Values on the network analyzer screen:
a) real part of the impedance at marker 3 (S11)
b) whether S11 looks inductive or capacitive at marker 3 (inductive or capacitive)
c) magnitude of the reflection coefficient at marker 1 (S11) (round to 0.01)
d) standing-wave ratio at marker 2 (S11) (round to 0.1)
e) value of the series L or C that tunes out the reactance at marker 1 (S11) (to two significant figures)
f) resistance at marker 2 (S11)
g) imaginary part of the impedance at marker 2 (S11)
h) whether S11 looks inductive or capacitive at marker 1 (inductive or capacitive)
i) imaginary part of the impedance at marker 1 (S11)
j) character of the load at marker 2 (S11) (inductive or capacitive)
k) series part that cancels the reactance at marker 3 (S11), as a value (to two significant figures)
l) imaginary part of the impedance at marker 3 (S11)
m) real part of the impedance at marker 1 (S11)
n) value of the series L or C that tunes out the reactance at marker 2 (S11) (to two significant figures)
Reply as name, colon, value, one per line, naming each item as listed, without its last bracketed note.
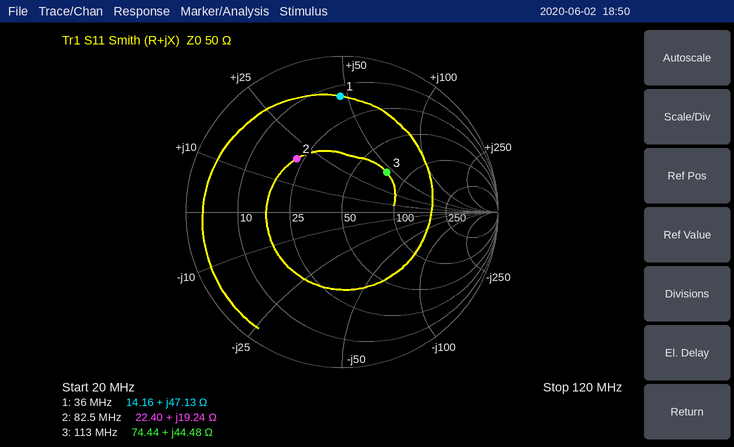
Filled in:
real part of the impedance at marker 3: 74.44 Ω
whether S11 looks inductive or capacitive at marker 3: inductive
magnitude of the reflection coefficient at marker 1 (S11): 0.74
standing-wave ratio at marker 2 (S11): 2.6
value of the series L or C that tunes out the reactance at marker 1 (S11): 94 pF
resistance at marker 2: 22.40 Ω
imaginary part of the impedance at marker 2: +19.24 Ω
whether S11 looks inductive or capacitive at marker 1: inductive
imaginary part of the impedance at marker 1: +47.13 Ω
character of the load at marker 2 (S11): inductive
series part that cancels the reactance at marker 3 (S11), as a value: 32 pF
imaginary part of the impedance at marker 3: +44.48 Ω
real part of the impedance at marker 1: 14.16 Ω
value of the series L or C that tunes out the reactance at marker 2 (S11): 100 pF
